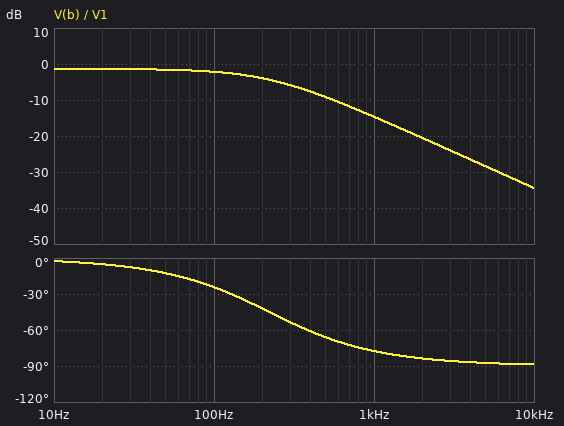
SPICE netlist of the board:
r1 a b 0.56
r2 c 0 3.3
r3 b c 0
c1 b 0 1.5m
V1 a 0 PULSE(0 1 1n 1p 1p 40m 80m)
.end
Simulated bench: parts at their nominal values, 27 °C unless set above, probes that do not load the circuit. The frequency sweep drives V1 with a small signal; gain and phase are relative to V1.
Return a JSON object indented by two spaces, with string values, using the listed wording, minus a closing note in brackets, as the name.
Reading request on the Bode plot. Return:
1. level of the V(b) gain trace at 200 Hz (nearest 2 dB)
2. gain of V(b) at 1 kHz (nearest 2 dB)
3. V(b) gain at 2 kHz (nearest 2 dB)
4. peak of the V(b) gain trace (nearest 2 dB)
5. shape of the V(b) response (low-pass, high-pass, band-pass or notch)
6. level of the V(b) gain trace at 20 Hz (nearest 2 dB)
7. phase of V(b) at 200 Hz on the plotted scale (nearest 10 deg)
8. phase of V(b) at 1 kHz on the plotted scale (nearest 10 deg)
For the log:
{
  "level of the V(b) gain trace at 200 Hz": "-4 dB",
  "gain of V(b) at 1 kHz": "-14 dB",
  "V(b) gain at 2 kHz": "-20 dB",
  "peak of the V(b) gain trace": "-2 dB",
  "shape of the V(b) response": "low-pass",
  "level of the V(b) gain trace at 20 Hz": "-2 dB",
  "phase of V(b) at 200 Hz on the plotted scale": "-40 deg",
  "phase of V(b) at 1 kHz on the plotted scale": "-80 deg"
}
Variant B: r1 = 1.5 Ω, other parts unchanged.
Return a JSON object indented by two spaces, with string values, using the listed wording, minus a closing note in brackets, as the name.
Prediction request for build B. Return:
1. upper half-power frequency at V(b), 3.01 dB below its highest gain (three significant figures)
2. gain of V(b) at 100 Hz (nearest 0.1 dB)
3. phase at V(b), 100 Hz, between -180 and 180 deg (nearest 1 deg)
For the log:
{
  "upper half-power frequency at V(b), 3.01 dB below its highest gain": "103 Hz",
  "gain of V(b) at 100 Hz": "-6.1 dB",
  "phase at V(b), 100 Hz, between -180 and 180 deg": "-44 deg"
}
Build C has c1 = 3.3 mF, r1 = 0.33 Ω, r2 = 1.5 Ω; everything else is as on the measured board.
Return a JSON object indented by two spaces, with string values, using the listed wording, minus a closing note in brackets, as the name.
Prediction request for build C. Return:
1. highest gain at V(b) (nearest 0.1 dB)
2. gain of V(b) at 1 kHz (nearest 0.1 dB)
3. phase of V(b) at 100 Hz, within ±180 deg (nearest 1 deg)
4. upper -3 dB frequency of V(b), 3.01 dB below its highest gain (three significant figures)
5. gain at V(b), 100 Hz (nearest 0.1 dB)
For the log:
{
  "highest gain at V(b)": "-1.7 dB",
  "gain of V(b) at 1 kHz": "-16.8 dB",
  "phase of V(b) at 100 Hz, within ±180 deg": "-29 deg",
  "upper -3 dB frequency of V(b), 3.01 dB below its highest gain": "178 Hz",
  "gain at V(b), 100 Hz": "-2.9 dB"
}
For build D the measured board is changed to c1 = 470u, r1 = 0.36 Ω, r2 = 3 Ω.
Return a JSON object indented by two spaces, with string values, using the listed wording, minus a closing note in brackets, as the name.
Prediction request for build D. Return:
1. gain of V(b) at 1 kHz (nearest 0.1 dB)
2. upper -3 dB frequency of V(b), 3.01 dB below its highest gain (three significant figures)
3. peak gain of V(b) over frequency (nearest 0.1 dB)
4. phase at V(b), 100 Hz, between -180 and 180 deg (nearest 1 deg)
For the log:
{
  "gain of V(b) at 1 kHz": "-3.8 dB",
  "upper -3 dB frequency of V(b), 3.01 dB below its highest gain": "1.05 kHz",
  "peak gain of V(b) over frequency": "-1.0 dB",
  "phase at V(b), 100 Hz, between -180 and 180 deg": "-5 deg"
}
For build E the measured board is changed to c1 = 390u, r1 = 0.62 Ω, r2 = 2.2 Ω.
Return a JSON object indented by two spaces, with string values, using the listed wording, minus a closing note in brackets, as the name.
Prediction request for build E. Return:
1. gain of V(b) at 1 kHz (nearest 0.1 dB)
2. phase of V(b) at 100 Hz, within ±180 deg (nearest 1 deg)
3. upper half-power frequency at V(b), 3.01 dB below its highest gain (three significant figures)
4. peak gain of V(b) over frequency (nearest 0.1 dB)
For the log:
{
  "gain of V(b) at 1 kHz": "-6.0 dB",
  "phase of V(b) at 100 Hz, within ±180 deg": "-7 deg",
  "upper half-power frequency at V(b), 3.01 dB below its highest gain": "844 Hz",
  "peak gain of V(b) over frequency": "-2.2 dB"
}
